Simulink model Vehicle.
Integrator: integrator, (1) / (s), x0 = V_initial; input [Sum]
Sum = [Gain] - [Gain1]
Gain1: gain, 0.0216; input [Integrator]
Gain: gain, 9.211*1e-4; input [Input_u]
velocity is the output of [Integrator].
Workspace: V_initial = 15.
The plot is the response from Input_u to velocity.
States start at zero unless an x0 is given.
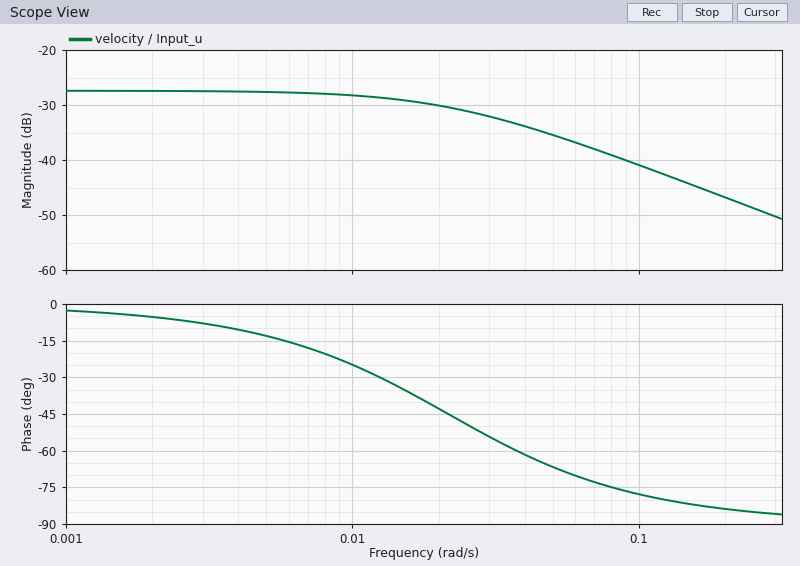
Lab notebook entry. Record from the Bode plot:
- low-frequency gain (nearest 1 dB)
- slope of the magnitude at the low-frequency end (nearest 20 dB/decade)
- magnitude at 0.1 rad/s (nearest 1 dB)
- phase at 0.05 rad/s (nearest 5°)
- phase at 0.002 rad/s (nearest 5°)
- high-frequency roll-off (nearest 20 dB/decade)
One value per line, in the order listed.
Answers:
-27 dB
0 dB/decade
-41 dB
-65°
-5°
-20 dB/decade
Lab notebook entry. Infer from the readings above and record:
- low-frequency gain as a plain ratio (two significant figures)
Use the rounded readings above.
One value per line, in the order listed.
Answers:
0.045
